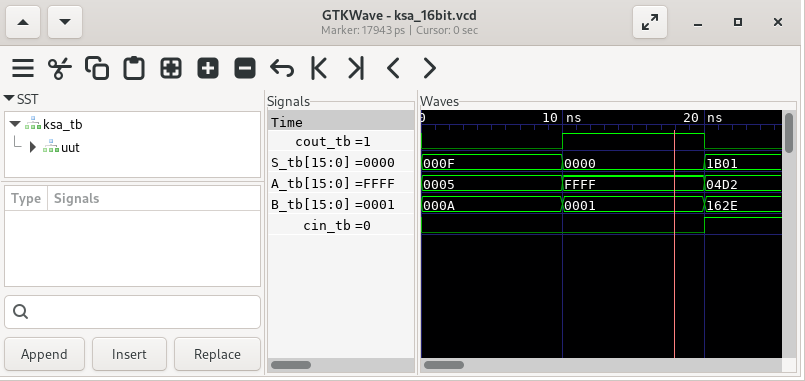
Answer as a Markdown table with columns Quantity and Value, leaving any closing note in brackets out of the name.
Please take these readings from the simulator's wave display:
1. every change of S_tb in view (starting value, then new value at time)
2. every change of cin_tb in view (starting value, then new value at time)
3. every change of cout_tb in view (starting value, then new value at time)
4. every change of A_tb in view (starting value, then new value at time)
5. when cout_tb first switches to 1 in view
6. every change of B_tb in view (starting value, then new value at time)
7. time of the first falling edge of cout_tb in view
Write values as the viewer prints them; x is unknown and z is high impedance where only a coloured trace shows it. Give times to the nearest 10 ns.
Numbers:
| Quantity | Value |
|---|---|
| every change of S_tb in view | 000F, 0000 at 10 ns, 1B01 at 20 ns |
| every change of cin_tb in view | 0, 1 at 20 ns |
| every change of cout_tb in view | 0, 1 at 10 ns, 0 at 20 ns |
| every change of A_tb in view | 0005, FFFF at 10 ns, 04D2 at 20 ns |
| when cout_tb first switches to 1 in view | 10 ns |
| every change of B_tb in view | 000A, 0001 at 10 ns, 162E at 20 ns |
| time of the first falling edge of cout_tb in view | 20 ns |
